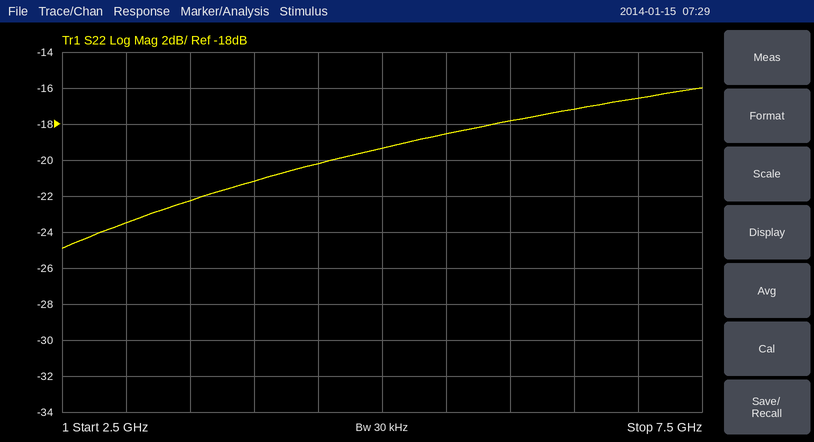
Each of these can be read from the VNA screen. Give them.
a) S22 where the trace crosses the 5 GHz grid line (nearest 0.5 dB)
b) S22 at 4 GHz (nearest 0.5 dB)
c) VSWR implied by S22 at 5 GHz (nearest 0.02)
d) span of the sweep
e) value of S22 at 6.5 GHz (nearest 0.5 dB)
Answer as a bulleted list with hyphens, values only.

- -19.5 dB
- -21.0 dB
- 1.24
- 5 GHz
- -17.0 dB
